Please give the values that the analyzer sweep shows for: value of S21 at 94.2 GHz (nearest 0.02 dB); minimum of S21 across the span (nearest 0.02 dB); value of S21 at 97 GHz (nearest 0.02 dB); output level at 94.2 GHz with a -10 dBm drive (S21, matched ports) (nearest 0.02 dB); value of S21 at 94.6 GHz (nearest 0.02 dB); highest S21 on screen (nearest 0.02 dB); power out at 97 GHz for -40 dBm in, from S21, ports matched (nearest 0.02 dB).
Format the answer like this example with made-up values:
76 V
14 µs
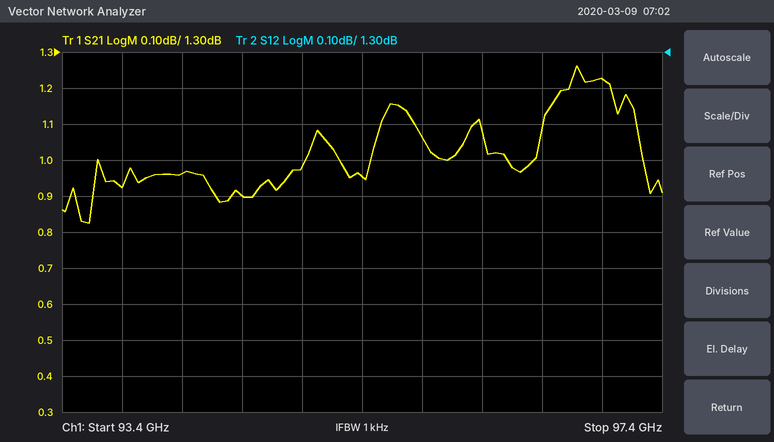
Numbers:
0.96 dB
0.82 dB
1.22 dB
-9.04 dBm
0.90 dB
1.26 dB
-38.78 dBm
